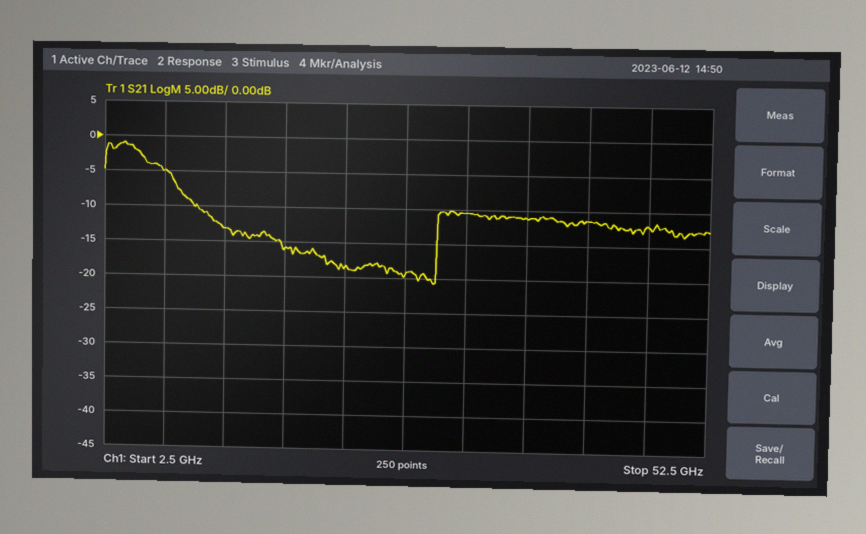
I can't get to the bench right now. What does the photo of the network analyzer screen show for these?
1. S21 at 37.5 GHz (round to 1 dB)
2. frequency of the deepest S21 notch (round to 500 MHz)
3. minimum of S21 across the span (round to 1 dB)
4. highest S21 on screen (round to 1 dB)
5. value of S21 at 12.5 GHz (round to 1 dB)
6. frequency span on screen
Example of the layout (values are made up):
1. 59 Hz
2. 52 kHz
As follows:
1. -11 dB
2. 30.0 GHz
3. -21 dB
4. -1 dB
5. -13 dB
6. 50 GHz
